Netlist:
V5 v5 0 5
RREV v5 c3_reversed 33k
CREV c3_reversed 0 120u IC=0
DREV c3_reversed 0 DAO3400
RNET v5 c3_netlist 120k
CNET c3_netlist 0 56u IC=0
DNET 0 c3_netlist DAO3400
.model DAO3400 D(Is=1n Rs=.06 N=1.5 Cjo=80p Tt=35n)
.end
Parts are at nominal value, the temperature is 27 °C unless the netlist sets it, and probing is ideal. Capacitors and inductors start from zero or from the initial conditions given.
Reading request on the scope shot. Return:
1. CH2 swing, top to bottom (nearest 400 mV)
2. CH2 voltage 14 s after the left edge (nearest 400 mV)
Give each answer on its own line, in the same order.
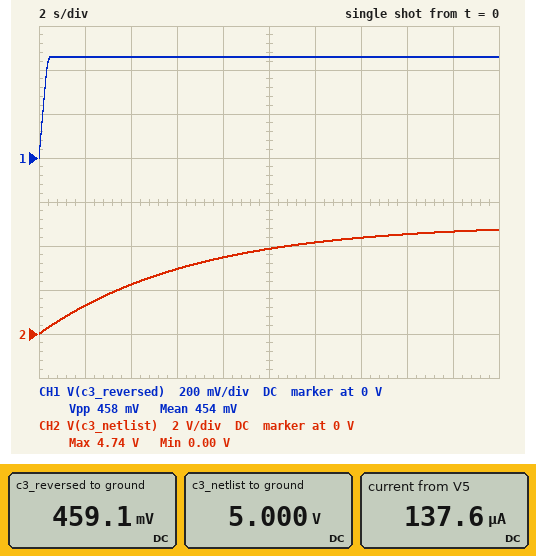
4.8 V
4.4 V
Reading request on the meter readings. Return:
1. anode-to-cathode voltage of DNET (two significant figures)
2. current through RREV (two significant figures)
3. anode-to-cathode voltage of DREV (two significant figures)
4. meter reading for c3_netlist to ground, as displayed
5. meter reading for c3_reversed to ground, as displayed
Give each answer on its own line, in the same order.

-5.0 V
140 µA
460 mV
5.000 V
459.1 mV
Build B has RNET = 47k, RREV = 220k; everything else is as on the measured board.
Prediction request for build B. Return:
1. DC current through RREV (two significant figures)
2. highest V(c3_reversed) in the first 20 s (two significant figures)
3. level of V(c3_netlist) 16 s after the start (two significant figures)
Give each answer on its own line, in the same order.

21 µA
390 mV
5.0 V
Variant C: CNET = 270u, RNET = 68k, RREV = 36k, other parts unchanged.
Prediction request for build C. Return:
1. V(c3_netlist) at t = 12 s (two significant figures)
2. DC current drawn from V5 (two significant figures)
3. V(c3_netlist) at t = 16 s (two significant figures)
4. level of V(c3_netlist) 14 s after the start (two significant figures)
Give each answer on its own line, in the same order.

2.4 V
130 µA
2.9 V
2.7 V
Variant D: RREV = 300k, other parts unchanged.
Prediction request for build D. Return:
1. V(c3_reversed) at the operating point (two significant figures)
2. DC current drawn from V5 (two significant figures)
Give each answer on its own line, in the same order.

370 mV
15 µA
